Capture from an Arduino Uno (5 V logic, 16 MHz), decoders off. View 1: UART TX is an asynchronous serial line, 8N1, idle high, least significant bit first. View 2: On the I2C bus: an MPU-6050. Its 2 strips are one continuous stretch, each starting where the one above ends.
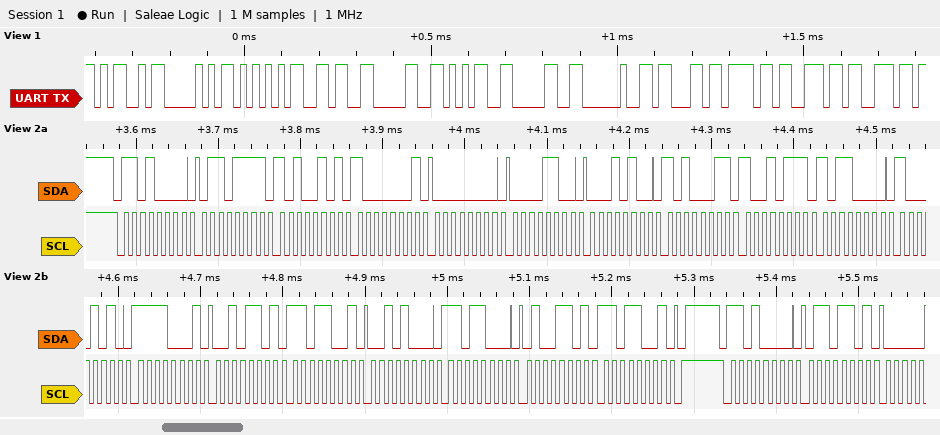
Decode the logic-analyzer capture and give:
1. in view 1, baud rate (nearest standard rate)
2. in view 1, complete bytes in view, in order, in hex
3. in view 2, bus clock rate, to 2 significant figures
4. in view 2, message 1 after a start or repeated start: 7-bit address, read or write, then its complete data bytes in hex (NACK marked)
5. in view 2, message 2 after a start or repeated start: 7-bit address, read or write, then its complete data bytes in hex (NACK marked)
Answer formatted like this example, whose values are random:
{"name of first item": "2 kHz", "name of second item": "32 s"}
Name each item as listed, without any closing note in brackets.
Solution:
{"in view 1, baud rate": "57600 baud", "in view 1, complete bytes in view, in order, in hex": "4D 50 55 36 30 35 30 20 63 6F 6E 6E", "in view 2, bus clock rate, to 2 significant figures": "100 kHz", "in view 2, message 1 after a start or repeated start: 7-bit address, read or write, then its complete data bytes in hex": "0x68 write: 6F A5 81 00 0C 14 A3 97 B0 8A F1 2D D9 28 D8 4D D9", "in view 2, message 2 after a start or repeated start: 7-bit address, read or write, then its complete data bytes in hex": "0x68 write: 6D"}
